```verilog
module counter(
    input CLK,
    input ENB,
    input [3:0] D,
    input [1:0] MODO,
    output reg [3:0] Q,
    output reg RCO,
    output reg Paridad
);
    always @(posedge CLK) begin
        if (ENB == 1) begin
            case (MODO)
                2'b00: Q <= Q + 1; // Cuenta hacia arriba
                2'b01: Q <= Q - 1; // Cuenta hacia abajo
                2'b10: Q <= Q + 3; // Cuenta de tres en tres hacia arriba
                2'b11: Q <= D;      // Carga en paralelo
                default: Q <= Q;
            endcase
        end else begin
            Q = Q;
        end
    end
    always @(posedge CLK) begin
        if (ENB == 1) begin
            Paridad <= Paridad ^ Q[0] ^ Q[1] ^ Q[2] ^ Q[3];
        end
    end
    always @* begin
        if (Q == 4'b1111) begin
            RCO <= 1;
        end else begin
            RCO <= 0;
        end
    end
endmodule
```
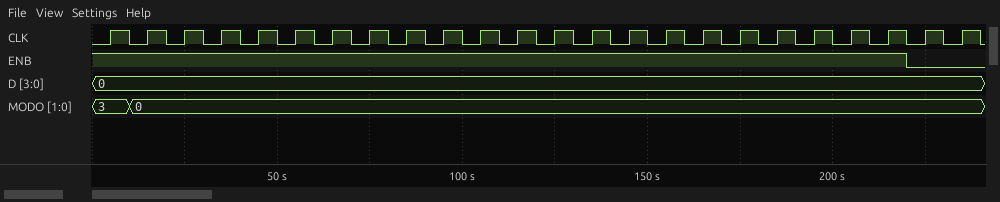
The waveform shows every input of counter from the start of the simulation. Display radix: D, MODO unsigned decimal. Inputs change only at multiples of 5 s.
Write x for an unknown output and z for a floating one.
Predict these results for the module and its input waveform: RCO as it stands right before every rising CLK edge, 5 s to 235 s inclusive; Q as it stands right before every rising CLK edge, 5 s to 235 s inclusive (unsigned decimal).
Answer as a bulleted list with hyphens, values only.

- x 0 0 0 0 0 0 0 0 0 0 0 0 0 0 0 1 0 0 0 0 0 0 0
- x, 0, 1, 2, 3, 4, 5, 6, 7, 8, 9, 10, 11, 12, 13, 14, 15, 0, 1, 2, 3, 4, 5, 5
